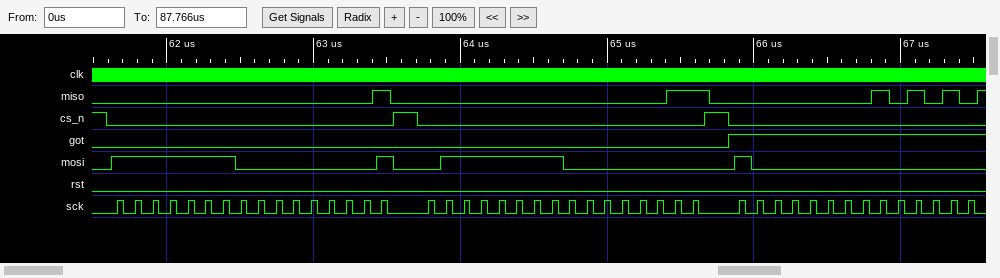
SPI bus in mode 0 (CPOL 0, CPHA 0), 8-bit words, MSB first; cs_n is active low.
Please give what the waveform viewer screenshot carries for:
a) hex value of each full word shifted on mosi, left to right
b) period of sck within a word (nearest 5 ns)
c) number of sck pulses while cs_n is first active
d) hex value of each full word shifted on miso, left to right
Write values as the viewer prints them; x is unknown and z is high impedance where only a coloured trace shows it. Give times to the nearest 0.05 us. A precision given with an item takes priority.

FE, 01, 7F, 00, 80
120 ns
16
00, 01, 00, 03, 00
